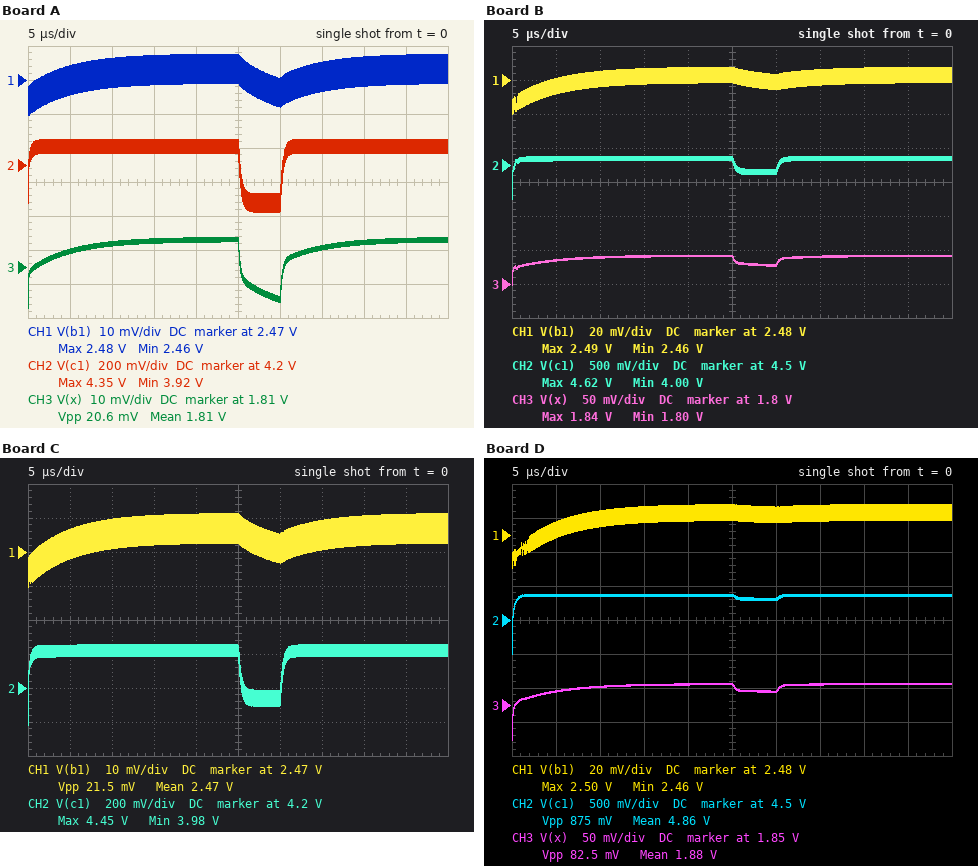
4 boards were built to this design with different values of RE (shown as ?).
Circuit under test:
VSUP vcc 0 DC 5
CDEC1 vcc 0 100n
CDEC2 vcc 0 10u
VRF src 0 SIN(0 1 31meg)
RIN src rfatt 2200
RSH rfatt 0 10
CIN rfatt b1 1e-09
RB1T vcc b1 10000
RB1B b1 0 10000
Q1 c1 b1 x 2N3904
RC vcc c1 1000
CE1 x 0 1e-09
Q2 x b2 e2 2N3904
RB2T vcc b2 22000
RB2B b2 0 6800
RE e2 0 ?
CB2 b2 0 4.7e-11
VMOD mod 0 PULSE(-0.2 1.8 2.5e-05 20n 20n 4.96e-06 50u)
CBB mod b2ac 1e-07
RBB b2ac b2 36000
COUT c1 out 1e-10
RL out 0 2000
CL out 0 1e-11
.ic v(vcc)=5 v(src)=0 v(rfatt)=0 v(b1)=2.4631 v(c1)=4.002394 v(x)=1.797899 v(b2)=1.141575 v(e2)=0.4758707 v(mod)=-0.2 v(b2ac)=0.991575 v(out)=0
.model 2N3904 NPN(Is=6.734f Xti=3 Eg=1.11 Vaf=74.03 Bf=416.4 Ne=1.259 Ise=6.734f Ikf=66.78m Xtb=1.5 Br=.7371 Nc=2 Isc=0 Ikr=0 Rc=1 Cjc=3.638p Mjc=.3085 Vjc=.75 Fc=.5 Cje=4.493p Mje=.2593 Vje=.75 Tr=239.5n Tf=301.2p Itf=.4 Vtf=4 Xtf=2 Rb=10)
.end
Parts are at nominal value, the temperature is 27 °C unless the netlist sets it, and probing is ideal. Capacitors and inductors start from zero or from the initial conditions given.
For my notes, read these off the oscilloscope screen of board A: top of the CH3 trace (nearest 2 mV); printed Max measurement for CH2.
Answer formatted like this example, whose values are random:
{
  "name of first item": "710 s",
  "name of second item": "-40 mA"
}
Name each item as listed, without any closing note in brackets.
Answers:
{
  "top of the CH3 trace": "1.818 V",
  "printed Max measurement for CH2": "4.35 V"
}
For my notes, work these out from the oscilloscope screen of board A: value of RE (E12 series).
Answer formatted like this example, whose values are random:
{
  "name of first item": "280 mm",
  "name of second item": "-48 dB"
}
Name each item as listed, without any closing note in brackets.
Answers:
{
  "value of RE": "680 Ω"
}
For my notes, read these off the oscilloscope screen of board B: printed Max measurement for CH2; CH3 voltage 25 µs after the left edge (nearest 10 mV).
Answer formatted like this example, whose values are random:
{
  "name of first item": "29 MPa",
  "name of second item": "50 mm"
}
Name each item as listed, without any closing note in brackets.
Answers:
{
  "printed Max measurement for CH2": "4.62 V",
  "CH3 voltage 25 µs after the left edge": "1.84 V"
}
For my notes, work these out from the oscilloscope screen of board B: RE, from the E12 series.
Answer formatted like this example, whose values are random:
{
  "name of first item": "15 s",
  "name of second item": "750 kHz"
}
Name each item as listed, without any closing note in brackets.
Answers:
{
  "RE, from the E12 series": "1.2 kΩ"
}
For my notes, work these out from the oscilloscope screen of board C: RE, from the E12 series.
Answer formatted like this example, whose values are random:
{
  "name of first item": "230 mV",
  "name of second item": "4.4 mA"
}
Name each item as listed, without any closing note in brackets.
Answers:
{
  "RE, from the E12 series": "820 Ω"
}
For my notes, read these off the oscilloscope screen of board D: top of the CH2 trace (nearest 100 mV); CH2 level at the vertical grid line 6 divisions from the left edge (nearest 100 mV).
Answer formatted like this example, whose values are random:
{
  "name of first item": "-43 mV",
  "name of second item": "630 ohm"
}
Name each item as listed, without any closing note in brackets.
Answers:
{
  "top of the CH2 trace": "4.9 V",
  "CH2 level at the vertical grid line 6 divisions from the left edge": "4.8 V"
}
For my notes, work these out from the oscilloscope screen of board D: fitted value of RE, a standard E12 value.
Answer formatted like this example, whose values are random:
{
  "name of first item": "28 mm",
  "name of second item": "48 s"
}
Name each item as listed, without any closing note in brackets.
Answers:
{
  "fitted value of RE, a standard E12 value": "3.9 kΩ"
}
